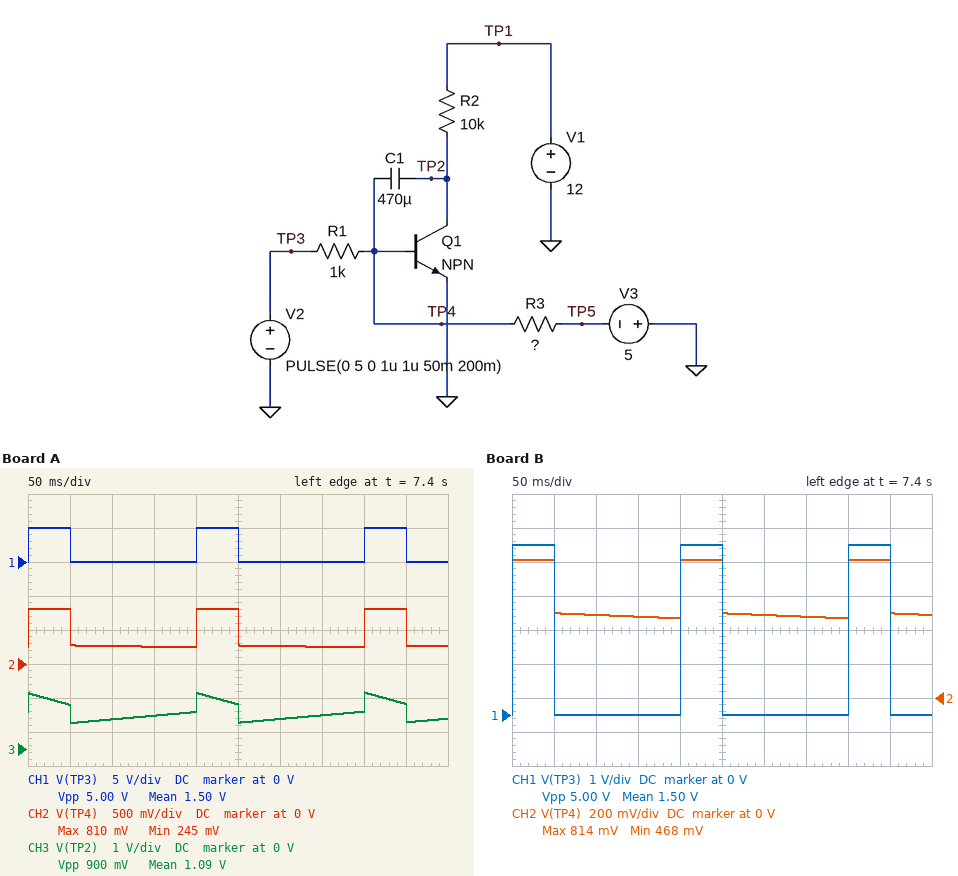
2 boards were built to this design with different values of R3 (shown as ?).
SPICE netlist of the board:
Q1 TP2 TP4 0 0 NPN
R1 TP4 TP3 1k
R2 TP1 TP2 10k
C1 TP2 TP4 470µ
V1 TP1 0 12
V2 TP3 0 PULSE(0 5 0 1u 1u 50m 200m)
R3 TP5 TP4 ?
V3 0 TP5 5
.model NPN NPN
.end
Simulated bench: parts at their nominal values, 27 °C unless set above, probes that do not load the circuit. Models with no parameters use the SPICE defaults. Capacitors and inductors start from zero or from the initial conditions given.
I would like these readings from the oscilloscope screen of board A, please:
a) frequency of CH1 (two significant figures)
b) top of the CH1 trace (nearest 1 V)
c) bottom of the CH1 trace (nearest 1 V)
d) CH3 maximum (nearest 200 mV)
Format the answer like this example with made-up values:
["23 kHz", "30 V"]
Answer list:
["5.0 Hz", "5 V", "0 V", "1.6 V"]
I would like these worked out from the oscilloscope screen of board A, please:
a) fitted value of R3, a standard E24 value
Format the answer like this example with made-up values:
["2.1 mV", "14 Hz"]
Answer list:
["6.2 kΩ"]
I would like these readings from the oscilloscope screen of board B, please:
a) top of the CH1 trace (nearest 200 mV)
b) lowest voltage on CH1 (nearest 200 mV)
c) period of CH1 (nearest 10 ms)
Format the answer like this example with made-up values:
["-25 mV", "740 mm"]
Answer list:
["5.0 V", "0 V", "200 ms"]
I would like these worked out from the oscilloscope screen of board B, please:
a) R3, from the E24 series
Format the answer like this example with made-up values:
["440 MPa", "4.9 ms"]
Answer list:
["8.2 kΩ"]
